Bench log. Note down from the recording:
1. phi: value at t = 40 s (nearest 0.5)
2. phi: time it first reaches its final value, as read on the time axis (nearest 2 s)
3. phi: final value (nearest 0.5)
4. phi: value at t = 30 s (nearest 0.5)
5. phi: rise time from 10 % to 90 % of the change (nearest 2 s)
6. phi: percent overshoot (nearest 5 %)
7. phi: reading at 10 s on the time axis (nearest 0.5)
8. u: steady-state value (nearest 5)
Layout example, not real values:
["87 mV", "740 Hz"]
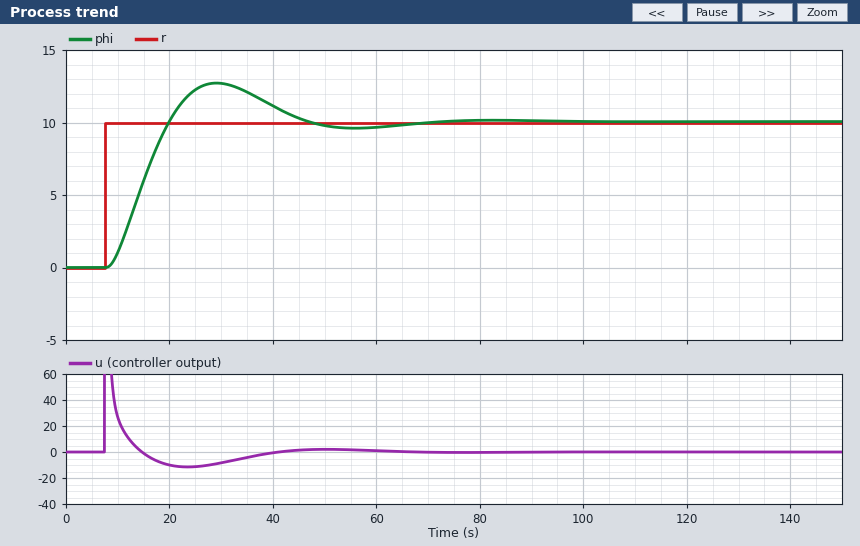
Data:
["11.0", "20 s", "10.0", "12.5", "8 s", "25 %", "1.0", "0"]
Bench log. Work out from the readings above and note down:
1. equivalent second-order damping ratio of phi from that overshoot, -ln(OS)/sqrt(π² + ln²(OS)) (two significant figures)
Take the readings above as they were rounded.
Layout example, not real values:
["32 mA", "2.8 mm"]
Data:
["0.40"]
